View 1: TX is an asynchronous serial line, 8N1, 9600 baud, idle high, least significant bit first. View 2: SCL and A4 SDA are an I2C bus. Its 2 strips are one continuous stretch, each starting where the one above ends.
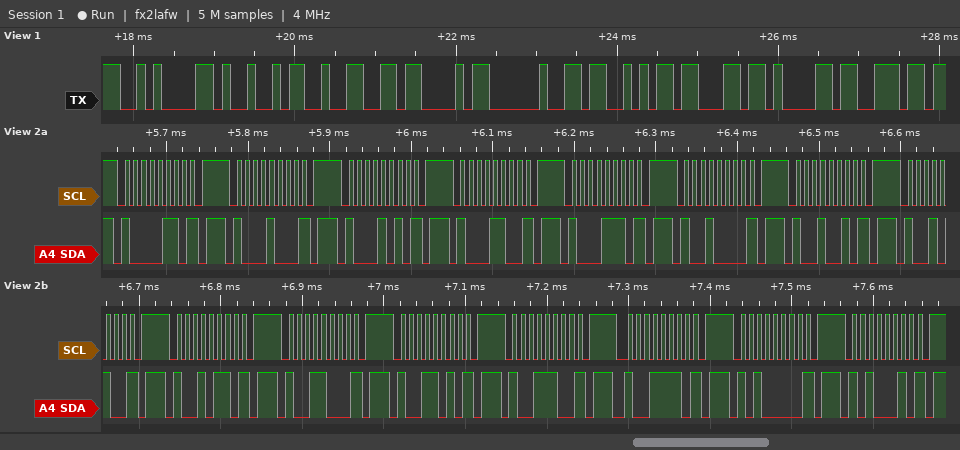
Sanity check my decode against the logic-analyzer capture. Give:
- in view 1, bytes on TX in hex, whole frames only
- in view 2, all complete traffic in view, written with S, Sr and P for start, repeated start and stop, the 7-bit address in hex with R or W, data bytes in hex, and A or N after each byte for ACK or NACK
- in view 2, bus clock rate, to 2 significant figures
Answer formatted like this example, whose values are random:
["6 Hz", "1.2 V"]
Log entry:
["0A 49 32 43 20 53 63 61 6E", "S 43W N P S 44W N P S 45W N P S 46W N P S 47W N P S 48W N P S 49W N P S 4AW N P S 4BW N P S 4CW N P S 4DW N P S 4EW N P S 4FW N P S 50W N P S 51W N P", "100 kHz"]
